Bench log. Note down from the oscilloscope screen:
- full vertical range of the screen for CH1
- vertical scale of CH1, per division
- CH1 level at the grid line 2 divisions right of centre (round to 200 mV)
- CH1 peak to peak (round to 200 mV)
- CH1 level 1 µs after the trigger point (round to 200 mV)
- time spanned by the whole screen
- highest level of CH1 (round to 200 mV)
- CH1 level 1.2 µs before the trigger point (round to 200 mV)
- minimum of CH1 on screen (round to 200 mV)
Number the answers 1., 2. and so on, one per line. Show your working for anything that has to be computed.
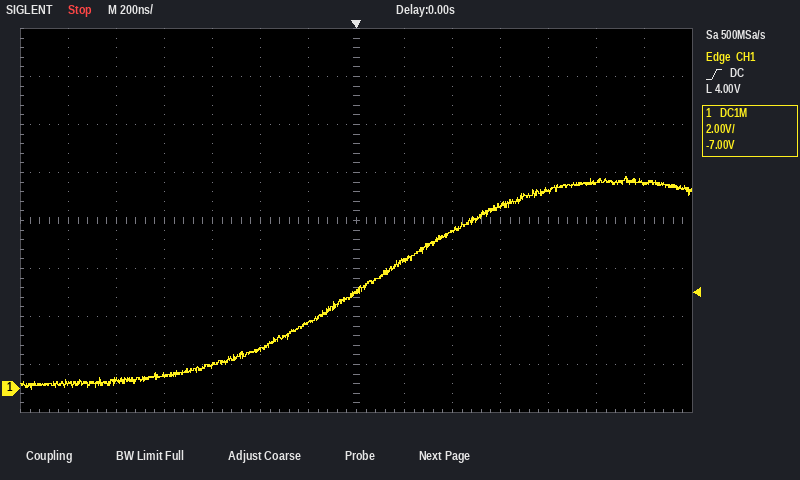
1. 16 V
2. 2 V
3. 6.6 V
4. 8.8 V − (0.0 V) = 8.8 V
5. 8.6 V
6. 2.8 µs
7. 8.8 V
8. 200 mV
9. 0.0 V
